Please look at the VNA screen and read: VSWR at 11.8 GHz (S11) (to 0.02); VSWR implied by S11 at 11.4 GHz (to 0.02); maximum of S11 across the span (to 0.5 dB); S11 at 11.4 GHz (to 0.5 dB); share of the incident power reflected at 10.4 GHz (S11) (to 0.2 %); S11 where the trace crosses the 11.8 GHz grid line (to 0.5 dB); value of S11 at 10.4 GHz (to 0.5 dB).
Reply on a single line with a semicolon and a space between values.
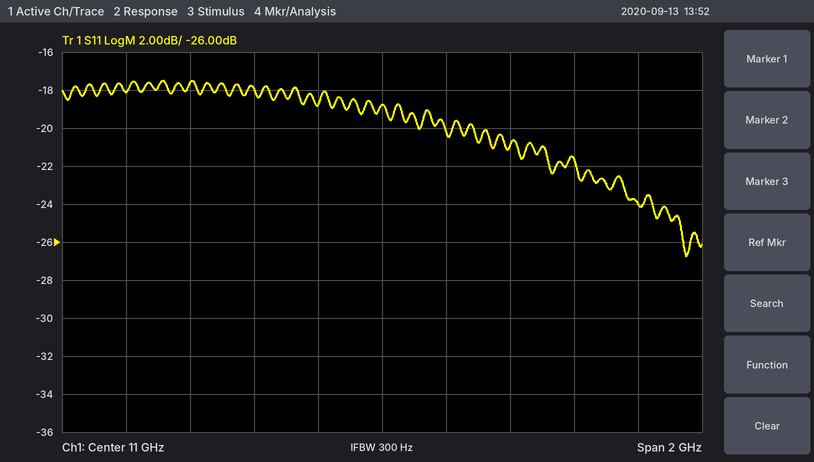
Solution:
1.14; 1.20; -17.5 dB; -21.0 dB; 1.8 %; -24.0 dB; -17.5 dB
